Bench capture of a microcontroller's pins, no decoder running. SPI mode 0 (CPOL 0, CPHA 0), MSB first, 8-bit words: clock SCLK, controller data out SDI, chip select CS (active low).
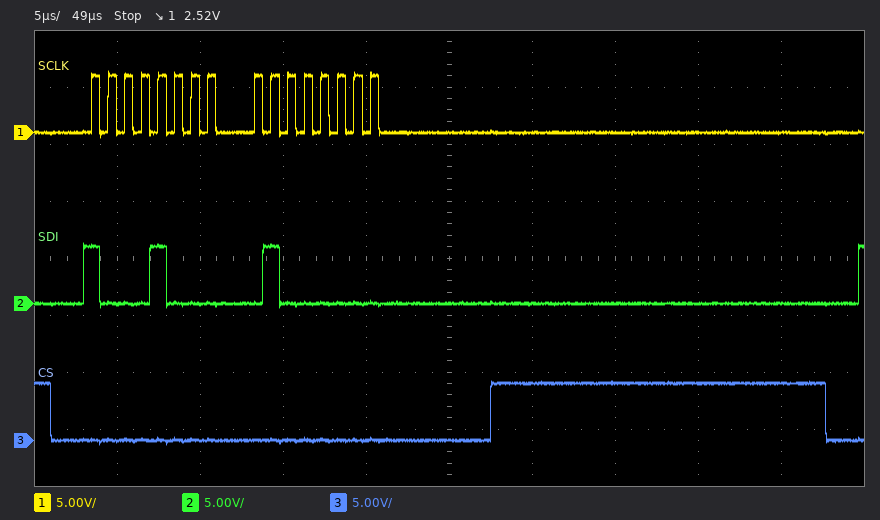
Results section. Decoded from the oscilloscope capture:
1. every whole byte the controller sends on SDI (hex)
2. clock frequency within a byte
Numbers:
0x88 0x40
1 MHz
